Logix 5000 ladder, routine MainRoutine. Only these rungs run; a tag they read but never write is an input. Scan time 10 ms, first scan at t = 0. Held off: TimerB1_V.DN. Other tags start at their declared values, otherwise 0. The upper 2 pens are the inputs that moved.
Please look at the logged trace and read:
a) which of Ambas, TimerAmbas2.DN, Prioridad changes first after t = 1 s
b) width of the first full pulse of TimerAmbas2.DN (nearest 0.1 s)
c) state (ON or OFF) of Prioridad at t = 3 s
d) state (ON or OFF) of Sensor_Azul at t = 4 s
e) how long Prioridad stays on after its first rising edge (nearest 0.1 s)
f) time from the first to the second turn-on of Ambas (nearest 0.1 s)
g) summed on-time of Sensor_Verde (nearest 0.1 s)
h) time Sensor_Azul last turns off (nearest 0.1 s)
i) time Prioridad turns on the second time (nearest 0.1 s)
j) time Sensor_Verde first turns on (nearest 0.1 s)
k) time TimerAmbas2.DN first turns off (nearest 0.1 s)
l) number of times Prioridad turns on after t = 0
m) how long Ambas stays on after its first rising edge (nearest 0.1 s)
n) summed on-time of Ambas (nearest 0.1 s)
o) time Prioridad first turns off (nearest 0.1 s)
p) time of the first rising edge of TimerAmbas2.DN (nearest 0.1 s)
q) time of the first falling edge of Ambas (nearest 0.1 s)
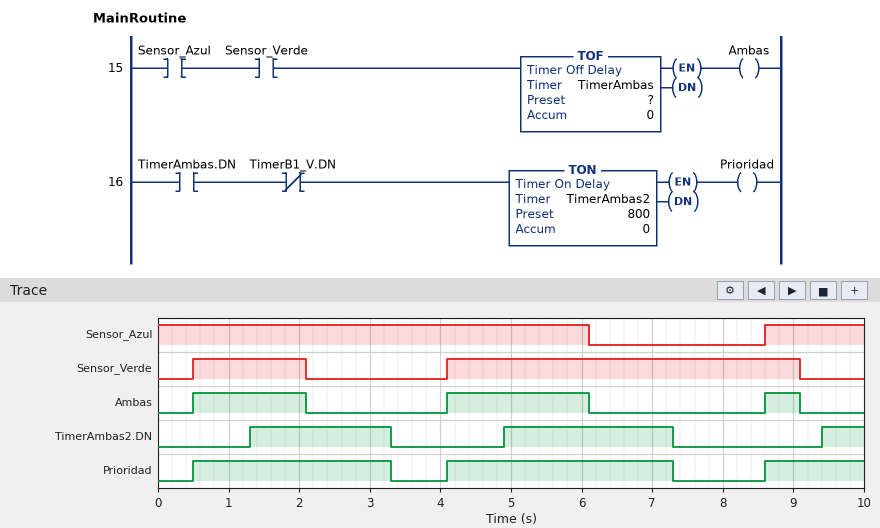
TimerAmbas2.DN
2.0 s
ON
ON
2.8 s
3.6 s
6.6 s
6.1 s
4.1 s
0.5 s
3.3 s
3
1.6 s
4.1 s
3.3 s
1.3 s
2.1 s
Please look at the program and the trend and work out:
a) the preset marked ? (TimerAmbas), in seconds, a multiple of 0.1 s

1.2 s
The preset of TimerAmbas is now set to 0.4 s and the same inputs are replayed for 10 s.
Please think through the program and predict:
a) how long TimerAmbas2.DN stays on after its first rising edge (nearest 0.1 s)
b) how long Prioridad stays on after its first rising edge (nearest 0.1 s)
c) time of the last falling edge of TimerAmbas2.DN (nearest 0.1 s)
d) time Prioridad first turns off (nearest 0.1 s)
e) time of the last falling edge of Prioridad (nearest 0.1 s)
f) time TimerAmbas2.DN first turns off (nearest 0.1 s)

1.2 s
2.0 s
9.5 s
2.5 s
9.5 s
2.5 s
